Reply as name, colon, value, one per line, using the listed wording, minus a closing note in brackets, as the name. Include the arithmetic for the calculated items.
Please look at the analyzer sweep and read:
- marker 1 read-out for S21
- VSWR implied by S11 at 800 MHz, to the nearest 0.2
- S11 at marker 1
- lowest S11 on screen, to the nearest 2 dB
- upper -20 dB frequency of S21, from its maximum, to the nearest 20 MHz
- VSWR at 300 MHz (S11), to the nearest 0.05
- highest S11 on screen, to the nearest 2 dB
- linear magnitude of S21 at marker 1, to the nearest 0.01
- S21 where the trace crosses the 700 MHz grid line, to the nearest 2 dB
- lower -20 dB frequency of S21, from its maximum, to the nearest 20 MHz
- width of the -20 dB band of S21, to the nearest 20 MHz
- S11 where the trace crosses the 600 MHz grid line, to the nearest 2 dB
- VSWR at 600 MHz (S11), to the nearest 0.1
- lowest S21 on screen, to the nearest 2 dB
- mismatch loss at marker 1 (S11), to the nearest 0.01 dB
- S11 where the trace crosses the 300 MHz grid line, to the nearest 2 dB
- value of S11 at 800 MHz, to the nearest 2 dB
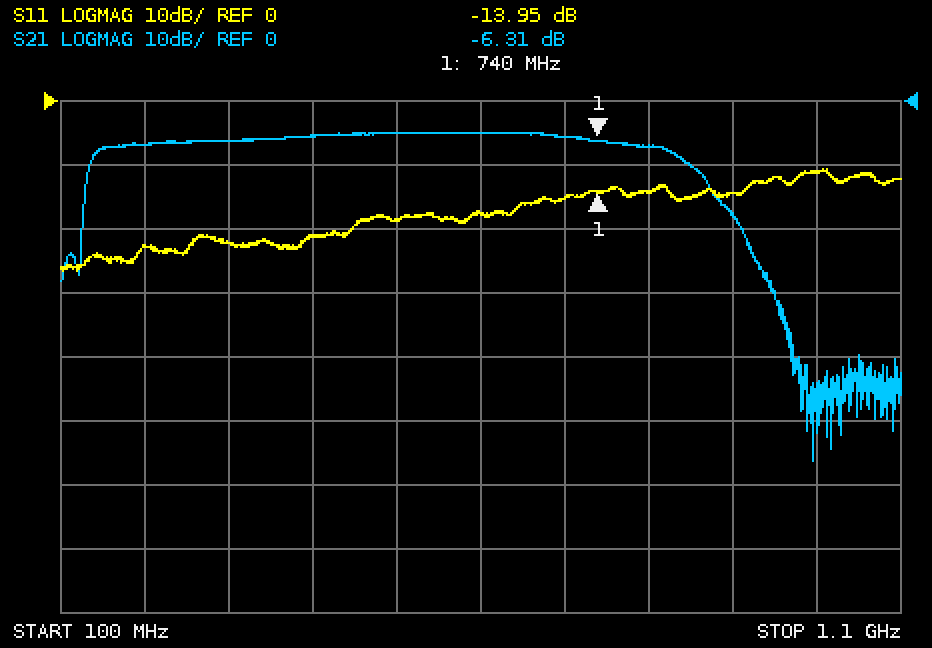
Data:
marker 1 read-out for S21: -6.31 dB
VSWR implied by S11 at 800 MHz, to the nearest 0.2: |Γ| = 10^(-14/20) = 0.1995; VSWR = (1 + 0.1995)/(1 − 0.1995) ≈ 1.50, so 1.4 to the nearest 0.2
S11 at marker 1: -13.95 dB
lowest S11 on screen, to the nearest 2 dB: -26 dB
upper -20 dB frequency of S21, from its maximum, to the nearest 20 MHz: 920 MHz
VSWR at 300 MHz (S11), to the nearest 0.05: |Γ| = 10^(-22/20) = 0.0794; VSWR = (1 + 0.0794)/(1 − 0.0794) ≈ 1.17, so 1.15 to the nearest 0.05
highest S11 on screen, to the nearest 2 dB: -10 dB
linear magnitude of S21 at marker 1, to the nearest 0.01: 10^(-6.31/20) ≈ 0.48
S21 where the trace crosses the 700 MHz grid line, to the nearest 2 dB: -6 dB
lower -20 dB frequency of S21, from its maximum, to the nearest 20 MHz: 120 MHz
width of the -20 dB band of S21, to the nearest 20 MHz: 920 MHz − 120 MHz = 800 MHz
S11 where the trace crosses the 600 MHz grid line, to the nearest 2 dB: -18 dB
VSWR at 600 MHz (S11), to the nearest 0.1: |Γ| = 10^(-18/20) = 0.1259; VSWR = (1 + 0.1259)/(1 − 0.1259) ≈ 1.3
lowest S21 on screen, to the nearest 2 dB: -56 dB
mismatch loss at marker 1 (S11), to the nearest 0.01 dB: −10 log10(1 − 10^(-13.95/10)) ≈ 0.18 dB
S11 where the trace crosses the 300 MHz grid line, to the nearest 2 dB: -22 dB
value of S11 at 800 MHz, to the nearest 2 dB: -14 dB
